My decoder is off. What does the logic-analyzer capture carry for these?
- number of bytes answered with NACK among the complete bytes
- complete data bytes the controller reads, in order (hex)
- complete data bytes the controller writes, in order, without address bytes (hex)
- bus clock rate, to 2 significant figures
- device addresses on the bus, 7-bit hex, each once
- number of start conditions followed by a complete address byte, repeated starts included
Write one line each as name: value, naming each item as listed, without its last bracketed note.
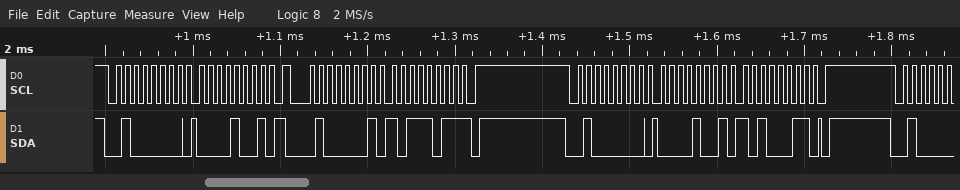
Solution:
number of bytes answered with NACK among the complete bytes: 1
complete data bytes the controller reads, in order: BB
complete data bytes the controller writes, in order, without address bytes: 09 09 A3
bus clock rate, to 2 significant figures: 100 kHz
device addresses on the bus, 7-bit hex, each once: 0x20
number of start conditions followed by a complete address byte, repeated starts included: 3
